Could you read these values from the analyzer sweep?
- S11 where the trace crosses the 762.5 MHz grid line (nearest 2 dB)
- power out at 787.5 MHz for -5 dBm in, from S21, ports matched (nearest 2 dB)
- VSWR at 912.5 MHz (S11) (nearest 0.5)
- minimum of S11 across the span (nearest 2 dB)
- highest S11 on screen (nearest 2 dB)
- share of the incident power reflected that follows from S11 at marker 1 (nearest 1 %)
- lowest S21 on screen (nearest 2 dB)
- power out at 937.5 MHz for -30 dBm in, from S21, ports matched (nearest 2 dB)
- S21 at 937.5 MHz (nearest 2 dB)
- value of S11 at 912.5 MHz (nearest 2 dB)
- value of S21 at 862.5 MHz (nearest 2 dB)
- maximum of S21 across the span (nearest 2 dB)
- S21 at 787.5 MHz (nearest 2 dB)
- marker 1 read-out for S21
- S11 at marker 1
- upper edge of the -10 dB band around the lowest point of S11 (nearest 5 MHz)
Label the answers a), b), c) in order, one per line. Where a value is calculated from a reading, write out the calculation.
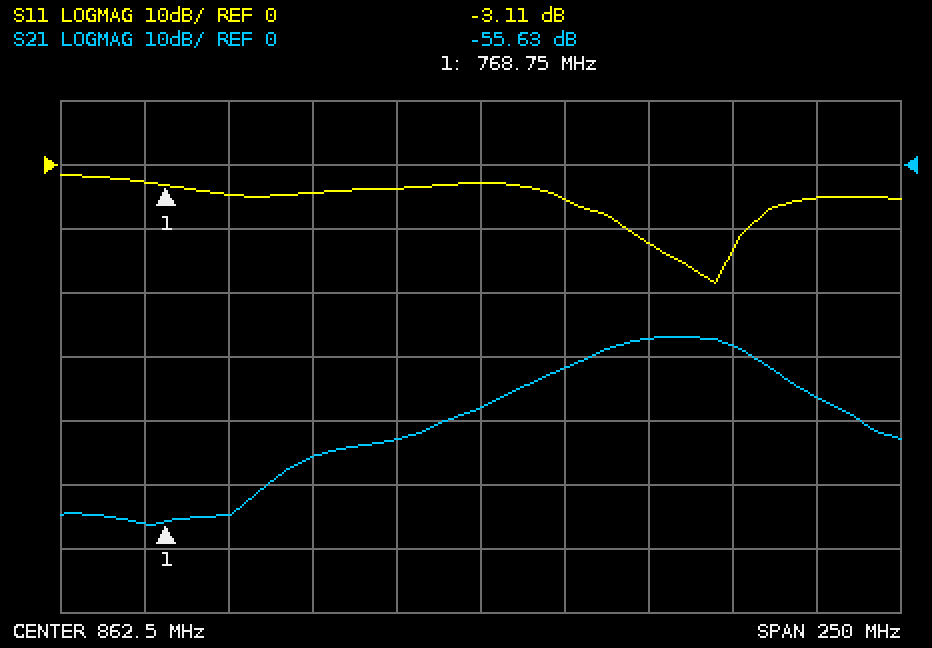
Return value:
a) -2 dB
b) -5 dBm + (-54 dB) = -60 dBm
c) |Γ| = 10^(-12/20) = 0.2512; VSWR = (1 + 0.2512)/(1 − 0.2512) ≈ 1.67, so 1.5 to the nearest 0.5
d) -18 dB
e) -2 dB
f) 10^(-3.11/10) ≈ 49 %
g) -56 dB
h) -30 dBm + (-28 dB) = -58 dBm
i) -28 dB
j) -12 dB
k) -38 dB
l) -26 dB
m) -54 dB
n) -55.63 dB
o) -3.11 dB
p) 940 MHz
